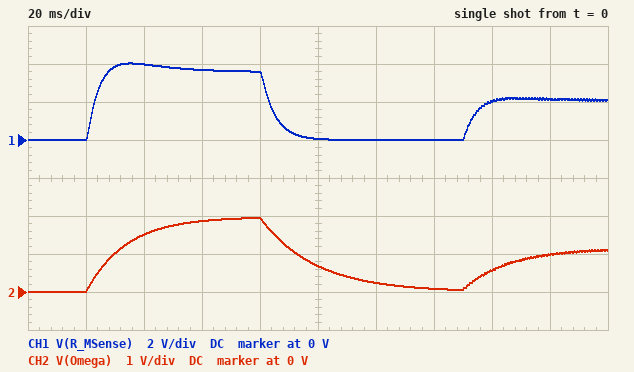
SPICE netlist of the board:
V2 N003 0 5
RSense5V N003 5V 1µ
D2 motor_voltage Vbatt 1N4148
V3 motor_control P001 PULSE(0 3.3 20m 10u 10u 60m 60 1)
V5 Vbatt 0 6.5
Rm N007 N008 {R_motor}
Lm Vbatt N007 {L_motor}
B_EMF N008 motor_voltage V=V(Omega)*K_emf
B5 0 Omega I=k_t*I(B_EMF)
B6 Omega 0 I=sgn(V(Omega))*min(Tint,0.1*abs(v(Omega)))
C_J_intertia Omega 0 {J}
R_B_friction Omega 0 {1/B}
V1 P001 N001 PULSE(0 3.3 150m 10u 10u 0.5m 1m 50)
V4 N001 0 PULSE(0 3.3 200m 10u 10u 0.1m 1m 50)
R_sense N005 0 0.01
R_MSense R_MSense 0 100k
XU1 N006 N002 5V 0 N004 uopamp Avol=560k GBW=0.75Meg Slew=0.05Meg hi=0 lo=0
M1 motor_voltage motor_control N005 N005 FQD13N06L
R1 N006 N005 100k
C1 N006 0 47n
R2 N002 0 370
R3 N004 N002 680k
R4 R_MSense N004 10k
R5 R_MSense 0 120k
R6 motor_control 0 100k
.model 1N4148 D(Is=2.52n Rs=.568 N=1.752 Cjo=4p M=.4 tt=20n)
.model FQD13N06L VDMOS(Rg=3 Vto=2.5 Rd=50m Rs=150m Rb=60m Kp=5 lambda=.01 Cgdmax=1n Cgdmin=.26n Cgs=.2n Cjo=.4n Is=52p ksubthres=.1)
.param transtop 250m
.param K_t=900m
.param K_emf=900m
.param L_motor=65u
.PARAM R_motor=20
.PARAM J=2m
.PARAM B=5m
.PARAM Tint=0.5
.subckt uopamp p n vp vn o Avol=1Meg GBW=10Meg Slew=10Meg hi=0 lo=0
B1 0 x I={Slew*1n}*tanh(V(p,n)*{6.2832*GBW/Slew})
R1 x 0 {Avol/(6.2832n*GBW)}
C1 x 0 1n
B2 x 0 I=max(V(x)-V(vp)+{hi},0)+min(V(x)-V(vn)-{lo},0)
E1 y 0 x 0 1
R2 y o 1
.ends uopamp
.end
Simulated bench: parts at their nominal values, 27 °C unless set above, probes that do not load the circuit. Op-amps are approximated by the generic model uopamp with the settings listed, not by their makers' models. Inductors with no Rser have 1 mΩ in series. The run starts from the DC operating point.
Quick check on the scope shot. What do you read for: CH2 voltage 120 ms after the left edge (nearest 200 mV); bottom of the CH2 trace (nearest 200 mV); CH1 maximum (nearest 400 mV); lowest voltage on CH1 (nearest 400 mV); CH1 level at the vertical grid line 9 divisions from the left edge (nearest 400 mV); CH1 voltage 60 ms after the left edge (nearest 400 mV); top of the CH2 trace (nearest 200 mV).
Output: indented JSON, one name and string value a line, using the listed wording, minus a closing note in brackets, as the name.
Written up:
{
  "CH2 voltage 120 ms after the left edge": "200 mV",
  "bottom of the CH2 trace": "0 V",
  "CH1 maximum": "4.0 V",
  "lowest voltage on CH1": "0 V",
  "CH1 level at the vertical grid line 9 divisions from the left edge": "2.0 V",
  "CH1 voltage 60 ms after the left edge": "3.6 V",
  "top of the CH2 trace": "2.0 V"
}
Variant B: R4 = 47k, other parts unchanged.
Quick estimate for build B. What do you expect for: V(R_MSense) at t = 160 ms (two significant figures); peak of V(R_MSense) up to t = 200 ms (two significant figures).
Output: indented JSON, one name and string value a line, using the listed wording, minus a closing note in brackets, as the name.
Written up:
{
  "V(R_MSense) at t = 160 ms": "1.3 V",
  "peak of V(R_MSense) up to t = 200 ms": "2.6 V"
}
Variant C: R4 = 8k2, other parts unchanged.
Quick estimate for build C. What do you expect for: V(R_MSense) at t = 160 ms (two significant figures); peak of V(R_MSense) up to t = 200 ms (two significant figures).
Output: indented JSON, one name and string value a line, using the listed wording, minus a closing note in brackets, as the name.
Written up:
{
  "V(R_MSense) at t = 160 ms": "2.1 V",
  "peak of V(R_MSense) up to t = 200 ms": "4.1 V"
}
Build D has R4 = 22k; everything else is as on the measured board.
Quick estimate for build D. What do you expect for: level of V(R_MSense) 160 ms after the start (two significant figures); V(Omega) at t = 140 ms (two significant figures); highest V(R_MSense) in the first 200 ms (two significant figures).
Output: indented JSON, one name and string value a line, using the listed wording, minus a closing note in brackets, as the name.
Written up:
{
  "level of V(R_MSense) 160 ms after the start": "1.7 V",
  "V(Omega) at t = 140 ms": "84 mV",
  "highest V(R_MSense) in the first 200 ms": "3.4 V"
}
